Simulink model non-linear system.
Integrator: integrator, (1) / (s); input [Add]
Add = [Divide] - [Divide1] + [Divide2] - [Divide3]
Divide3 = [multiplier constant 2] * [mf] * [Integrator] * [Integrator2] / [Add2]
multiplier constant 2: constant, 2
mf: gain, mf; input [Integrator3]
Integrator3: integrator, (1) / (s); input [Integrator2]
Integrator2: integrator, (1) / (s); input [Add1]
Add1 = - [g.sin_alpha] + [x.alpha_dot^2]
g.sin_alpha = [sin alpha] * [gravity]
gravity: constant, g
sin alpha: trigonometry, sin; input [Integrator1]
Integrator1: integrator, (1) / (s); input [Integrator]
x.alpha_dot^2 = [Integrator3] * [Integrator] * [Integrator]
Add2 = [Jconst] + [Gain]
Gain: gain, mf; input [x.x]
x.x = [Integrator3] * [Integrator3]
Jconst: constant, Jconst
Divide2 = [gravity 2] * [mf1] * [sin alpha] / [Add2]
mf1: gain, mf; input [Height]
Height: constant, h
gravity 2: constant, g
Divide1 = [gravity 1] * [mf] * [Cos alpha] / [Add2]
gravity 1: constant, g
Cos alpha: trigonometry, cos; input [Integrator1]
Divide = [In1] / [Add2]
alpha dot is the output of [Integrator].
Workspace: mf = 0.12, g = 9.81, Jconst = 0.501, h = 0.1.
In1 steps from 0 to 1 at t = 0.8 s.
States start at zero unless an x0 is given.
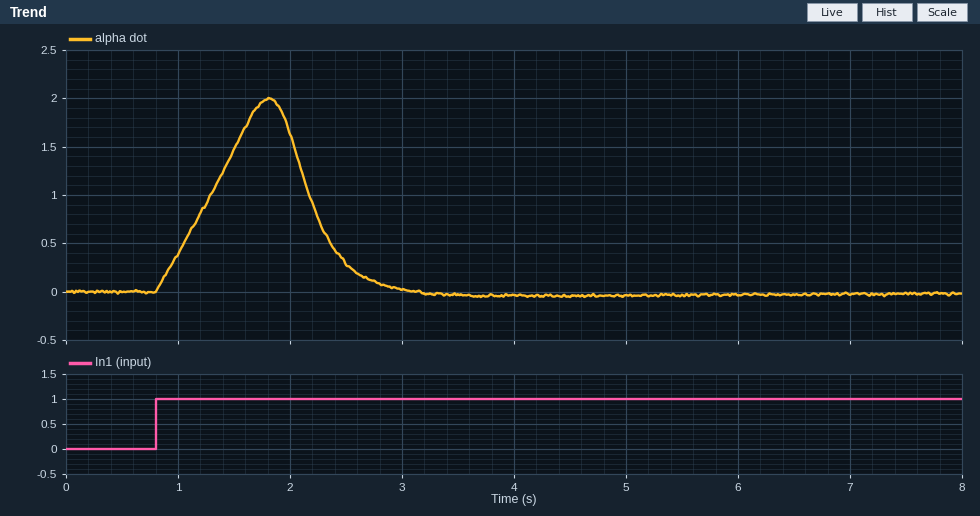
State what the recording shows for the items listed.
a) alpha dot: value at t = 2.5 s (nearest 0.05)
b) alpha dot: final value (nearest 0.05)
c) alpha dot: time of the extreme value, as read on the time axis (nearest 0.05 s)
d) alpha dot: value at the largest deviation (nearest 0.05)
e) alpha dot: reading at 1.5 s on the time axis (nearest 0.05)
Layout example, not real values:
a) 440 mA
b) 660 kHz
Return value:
a) 0.30
b) 0.00
c) 1.80 s
d) 2.00
e) 1.45
